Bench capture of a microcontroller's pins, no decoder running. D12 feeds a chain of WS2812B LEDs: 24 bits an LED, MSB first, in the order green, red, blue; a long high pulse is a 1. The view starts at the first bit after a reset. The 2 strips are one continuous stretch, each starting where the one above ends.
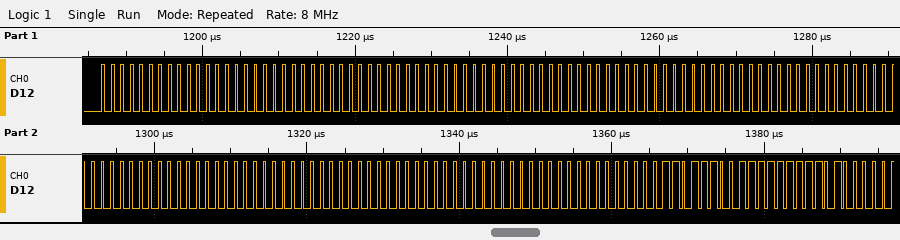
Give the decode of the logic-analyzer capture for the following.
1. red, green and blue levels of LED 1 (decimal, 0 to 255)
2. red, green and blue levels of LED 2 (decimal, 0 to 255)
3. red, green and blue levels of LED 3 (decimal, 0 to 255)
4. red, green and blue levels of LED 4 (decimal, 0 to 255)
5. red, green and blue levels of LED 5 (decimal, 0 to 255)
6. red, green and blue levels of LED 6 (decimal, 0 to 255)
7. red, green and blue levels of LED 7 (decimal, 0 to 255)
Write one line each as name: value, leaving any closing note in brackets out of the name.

red, green and blue levels of LED 1: 0, 0, 0
red, green and blue levels of LED 2: 0, 0, 0
red, green and blue levels of LED 3: 0, 0, 0
red, green and blue levels of LED 4: 0, 0, 0
red, green and blue levels of LED 5: 0, 0, 0
red, green and blue levels of LED 6: 0, 0, 0
red, green and blue levels of LED 7: 255, 220, 160
